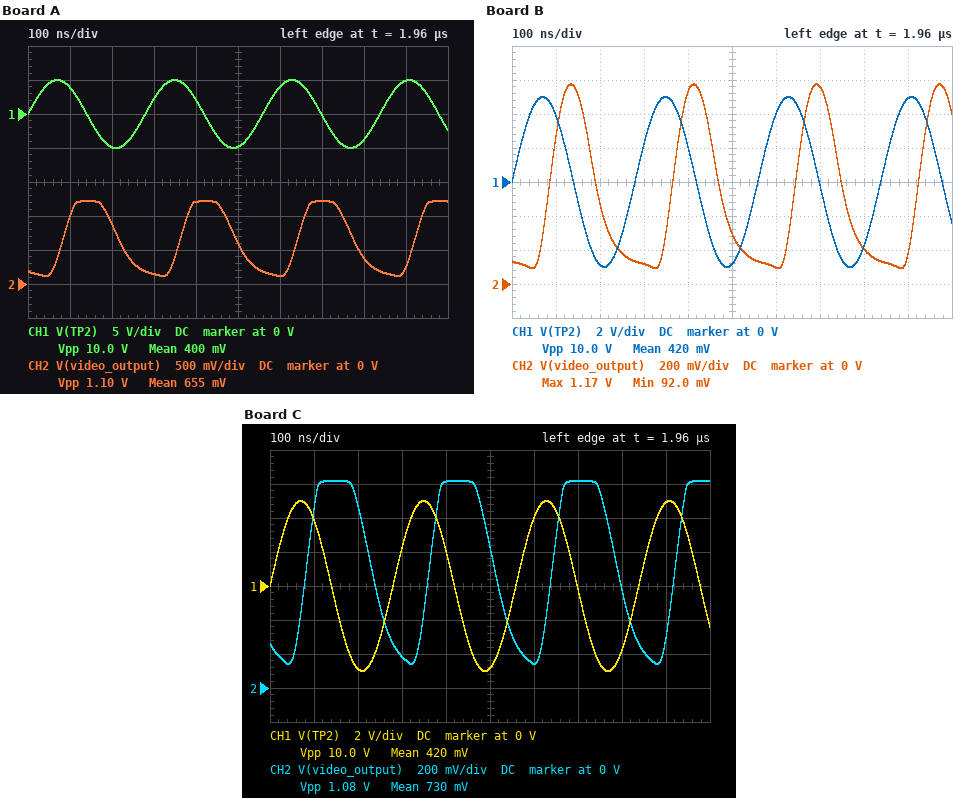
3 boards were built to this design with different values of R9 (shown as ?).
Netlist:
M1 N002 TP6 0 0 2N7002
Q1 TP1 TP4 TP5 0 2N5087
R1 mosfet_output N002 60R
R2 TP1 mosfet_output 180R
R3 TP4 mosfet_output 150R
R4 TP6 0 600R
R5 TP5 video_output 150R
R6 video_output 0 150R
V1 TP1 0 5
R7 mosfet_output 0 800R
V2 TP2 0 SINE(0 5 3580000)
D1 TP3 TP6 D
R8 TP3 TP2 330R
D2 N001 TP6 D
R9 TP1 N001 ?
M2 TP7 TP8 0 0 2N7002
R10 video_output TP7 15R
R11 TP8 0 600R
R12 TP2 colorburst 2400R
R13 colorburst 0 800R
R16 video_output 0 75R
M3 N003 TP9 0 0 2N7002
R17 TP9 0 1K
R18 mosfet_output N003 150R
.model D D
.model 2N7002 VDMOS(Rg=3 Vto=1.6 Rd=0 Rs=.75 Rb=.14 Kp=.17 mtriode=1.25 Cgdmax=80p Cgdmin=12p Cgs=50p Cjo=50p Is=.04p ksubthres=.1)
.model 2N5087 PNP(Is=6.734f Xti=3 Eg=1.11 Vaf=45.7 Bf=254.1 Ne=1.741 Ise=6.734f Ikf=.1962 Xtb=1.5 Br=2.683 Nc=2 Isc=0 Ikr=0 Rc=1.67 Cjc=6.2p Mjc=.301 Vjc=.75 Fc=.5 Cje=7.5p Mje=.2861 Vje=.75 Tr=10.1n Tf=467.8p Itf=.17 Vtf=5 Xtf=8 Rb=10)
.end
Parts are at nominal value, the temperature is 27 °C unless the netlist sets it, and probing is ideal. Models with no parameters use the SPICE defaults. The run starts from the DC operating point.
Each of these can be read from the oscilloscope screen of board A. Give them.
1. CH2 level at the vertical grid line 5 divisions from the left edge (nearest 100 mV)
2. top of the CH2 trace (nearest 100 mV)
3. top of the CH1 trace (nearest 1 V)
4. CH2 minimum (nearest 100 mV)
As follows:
600 mV
1.2 V
5 V
100 mV
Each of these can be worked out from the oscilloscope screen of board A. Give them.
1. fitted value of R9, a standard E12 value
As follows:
1.8 kΩ
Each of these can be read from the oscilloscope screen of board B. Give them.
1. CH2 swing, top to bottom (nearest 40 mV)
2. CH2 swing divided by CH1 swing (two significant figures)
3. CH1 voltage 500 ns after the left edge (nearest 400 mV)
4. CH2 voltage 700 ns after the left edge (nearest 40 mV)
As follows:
1.08 V
0.11
-4.8 V
1.16 V
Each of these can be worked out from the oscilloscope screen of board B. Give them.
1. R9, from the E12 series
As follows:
3.3 kΩ
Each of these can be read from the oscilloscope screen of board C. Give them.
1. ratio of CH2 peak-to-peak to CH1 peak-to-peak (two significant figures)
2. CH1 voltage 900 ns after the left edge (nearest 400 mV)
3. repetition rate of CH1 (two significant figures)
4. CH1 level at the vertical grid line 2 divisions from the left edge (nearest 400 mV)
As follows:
0.11
4.8 V
3.6 MHz
-4.8 V
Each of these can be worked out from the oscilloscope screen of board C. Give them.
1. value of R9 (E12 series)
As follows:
1.5 kΩ
